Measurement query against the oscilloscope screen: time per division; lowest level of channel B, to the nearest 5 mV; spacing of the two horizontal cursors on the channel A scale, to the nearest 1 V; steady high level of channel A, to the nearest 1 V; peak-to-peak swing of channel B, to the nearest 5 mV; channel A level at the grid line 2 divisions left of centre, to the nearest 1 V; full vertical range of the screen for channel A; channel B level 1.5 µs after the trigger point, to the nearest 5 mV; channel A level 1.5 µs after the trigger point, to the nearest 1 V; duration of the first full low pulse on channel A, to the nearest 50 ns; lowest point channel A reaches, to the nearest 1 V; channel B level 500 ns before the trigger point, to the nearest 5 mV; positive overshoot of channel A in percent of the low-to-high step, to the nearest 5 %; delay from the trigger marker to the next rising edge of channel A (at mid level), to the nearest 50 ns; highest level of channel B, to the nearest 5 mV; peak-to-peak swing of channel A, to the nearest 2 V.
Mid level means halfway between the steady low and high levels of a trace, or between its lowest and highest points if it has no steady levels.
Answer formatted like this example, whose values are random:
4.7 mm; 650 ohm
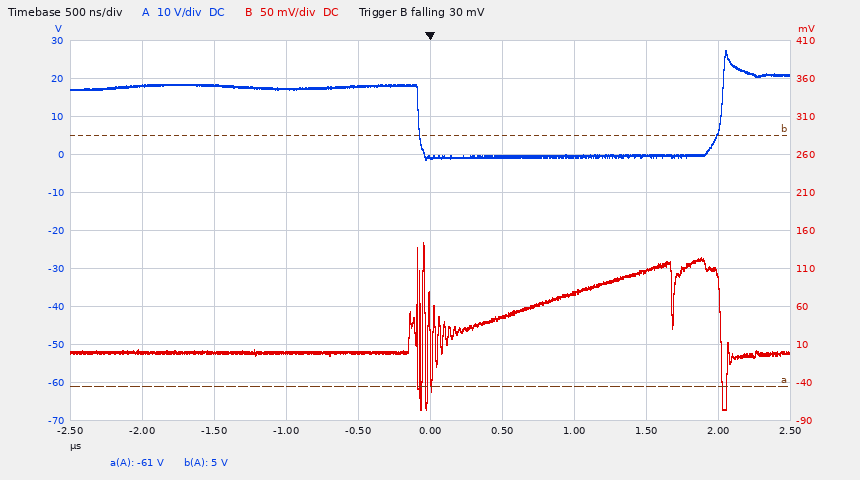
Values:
500 ns; -75 mV; 66 V; 18 V; 220 mV; 17 V; 100 V; 105 mV; 0 V; 2.10 µs; -1 V; 0 mV; 50 %; 2.00 µs; 145 mV; 28 V
